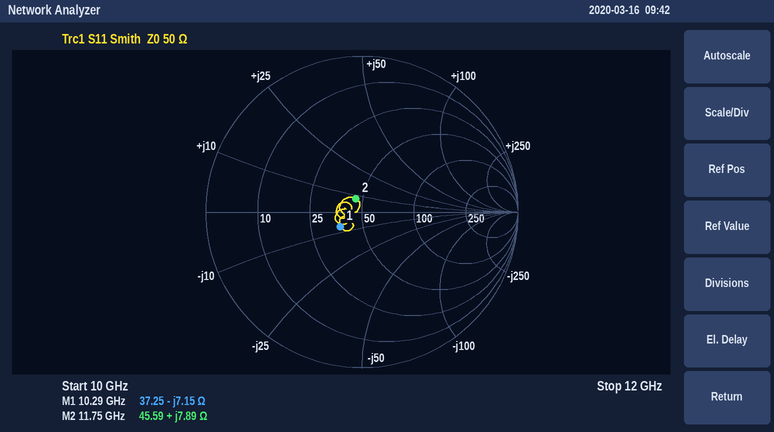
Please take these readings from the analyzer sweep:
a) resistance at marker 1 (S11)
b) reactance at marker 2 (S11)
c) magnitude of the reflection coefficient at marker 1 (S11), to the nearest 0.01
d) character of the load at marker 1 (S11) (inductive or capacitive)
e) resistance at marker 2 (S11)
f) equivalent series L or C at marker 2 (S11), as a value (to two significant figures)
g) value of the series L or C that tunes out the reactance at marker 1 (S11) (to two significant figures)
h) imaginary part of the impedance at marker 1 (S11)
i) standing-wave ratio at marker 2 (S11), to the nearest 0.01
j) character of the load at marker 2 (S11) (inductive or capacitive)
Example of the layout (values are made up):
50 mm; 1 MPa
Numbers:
37.25 Ω; +7.89 Ω; 0.17; capacitive; 45.59 Ω; 110 pH; 110 pH; -7.15 Ω; 1.21; inductive
